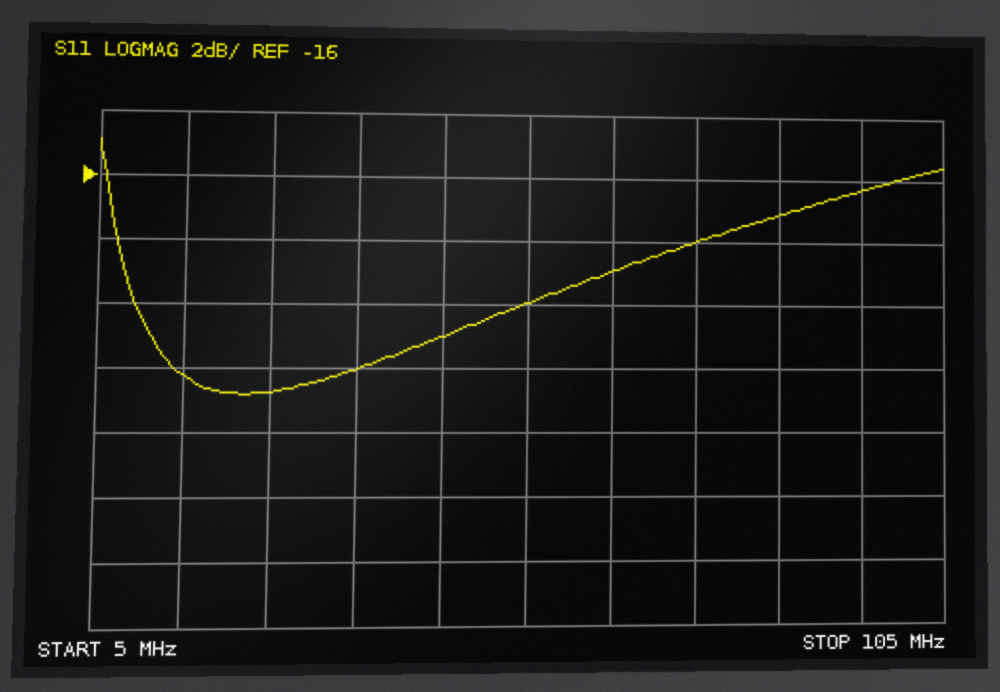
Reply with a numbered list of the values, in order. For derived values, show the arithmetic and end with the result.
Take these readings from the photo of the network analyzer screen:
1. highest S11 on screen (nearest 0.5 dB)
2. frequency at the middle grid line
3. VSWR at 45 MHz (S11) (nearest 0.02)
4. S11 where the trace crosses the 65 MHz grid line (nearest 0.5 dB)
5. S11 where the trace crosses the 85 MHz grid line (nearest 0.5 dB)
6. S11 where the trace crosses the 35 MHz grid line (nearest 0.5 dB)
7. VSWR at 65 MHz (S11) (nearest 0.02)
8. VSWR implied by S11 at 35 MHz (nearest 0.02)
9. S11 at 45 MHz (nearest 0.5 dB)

1. -15.0 dB
2. 55 MHz
3. |Γ| = 10^(-21/20) = 0.0891; VSWR = (1 + 0.0891)/(1 − 0.0891) ≈ 1.20
4. -19.0 dB
5. -17.0 dB
6. -22.0 dB
7. |Γ| = 10^(-19/20) = 0.1122; VSWR = (1 + 0.1122)/(1 − 0.1122) ≈ 1.25, so 1.26 to the nearest 0.02
8. |Γ| = 10^(-22/20) = 0.0794; VSWR = (1 + 0.0794)/(1 − 0.0794) ≈ 1.17, so 1.18 to the nearest 0.02
9. -21.0 dB
